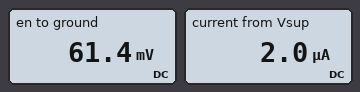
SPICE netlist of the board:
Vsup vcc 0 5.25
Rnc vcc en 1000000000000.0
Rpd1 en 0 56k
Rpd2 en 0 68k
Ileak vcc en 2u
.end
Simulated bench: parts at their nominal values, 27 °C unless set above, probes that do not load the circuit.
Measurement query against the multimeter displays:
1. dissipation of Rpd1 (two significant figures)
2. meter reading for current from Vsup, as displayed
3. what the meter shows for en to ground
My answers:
67 nW
2.0 µA
61.4 mV
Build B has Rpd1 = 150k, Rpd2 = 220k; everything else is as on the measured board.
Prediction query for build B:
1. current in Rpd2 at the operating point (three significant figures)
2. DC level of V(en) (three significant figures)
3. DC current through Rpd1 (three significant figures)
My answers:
811 nA
178 mV
1.19 µA
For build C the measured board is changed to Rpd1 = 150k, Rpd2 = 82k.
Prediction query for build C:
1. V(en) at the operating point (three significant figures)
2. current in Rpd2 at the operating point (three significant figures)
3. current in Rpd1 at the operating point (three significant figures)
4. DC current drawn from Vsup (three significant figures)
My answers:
106 mV
1.29 µA
707 nA
2.00 µA
